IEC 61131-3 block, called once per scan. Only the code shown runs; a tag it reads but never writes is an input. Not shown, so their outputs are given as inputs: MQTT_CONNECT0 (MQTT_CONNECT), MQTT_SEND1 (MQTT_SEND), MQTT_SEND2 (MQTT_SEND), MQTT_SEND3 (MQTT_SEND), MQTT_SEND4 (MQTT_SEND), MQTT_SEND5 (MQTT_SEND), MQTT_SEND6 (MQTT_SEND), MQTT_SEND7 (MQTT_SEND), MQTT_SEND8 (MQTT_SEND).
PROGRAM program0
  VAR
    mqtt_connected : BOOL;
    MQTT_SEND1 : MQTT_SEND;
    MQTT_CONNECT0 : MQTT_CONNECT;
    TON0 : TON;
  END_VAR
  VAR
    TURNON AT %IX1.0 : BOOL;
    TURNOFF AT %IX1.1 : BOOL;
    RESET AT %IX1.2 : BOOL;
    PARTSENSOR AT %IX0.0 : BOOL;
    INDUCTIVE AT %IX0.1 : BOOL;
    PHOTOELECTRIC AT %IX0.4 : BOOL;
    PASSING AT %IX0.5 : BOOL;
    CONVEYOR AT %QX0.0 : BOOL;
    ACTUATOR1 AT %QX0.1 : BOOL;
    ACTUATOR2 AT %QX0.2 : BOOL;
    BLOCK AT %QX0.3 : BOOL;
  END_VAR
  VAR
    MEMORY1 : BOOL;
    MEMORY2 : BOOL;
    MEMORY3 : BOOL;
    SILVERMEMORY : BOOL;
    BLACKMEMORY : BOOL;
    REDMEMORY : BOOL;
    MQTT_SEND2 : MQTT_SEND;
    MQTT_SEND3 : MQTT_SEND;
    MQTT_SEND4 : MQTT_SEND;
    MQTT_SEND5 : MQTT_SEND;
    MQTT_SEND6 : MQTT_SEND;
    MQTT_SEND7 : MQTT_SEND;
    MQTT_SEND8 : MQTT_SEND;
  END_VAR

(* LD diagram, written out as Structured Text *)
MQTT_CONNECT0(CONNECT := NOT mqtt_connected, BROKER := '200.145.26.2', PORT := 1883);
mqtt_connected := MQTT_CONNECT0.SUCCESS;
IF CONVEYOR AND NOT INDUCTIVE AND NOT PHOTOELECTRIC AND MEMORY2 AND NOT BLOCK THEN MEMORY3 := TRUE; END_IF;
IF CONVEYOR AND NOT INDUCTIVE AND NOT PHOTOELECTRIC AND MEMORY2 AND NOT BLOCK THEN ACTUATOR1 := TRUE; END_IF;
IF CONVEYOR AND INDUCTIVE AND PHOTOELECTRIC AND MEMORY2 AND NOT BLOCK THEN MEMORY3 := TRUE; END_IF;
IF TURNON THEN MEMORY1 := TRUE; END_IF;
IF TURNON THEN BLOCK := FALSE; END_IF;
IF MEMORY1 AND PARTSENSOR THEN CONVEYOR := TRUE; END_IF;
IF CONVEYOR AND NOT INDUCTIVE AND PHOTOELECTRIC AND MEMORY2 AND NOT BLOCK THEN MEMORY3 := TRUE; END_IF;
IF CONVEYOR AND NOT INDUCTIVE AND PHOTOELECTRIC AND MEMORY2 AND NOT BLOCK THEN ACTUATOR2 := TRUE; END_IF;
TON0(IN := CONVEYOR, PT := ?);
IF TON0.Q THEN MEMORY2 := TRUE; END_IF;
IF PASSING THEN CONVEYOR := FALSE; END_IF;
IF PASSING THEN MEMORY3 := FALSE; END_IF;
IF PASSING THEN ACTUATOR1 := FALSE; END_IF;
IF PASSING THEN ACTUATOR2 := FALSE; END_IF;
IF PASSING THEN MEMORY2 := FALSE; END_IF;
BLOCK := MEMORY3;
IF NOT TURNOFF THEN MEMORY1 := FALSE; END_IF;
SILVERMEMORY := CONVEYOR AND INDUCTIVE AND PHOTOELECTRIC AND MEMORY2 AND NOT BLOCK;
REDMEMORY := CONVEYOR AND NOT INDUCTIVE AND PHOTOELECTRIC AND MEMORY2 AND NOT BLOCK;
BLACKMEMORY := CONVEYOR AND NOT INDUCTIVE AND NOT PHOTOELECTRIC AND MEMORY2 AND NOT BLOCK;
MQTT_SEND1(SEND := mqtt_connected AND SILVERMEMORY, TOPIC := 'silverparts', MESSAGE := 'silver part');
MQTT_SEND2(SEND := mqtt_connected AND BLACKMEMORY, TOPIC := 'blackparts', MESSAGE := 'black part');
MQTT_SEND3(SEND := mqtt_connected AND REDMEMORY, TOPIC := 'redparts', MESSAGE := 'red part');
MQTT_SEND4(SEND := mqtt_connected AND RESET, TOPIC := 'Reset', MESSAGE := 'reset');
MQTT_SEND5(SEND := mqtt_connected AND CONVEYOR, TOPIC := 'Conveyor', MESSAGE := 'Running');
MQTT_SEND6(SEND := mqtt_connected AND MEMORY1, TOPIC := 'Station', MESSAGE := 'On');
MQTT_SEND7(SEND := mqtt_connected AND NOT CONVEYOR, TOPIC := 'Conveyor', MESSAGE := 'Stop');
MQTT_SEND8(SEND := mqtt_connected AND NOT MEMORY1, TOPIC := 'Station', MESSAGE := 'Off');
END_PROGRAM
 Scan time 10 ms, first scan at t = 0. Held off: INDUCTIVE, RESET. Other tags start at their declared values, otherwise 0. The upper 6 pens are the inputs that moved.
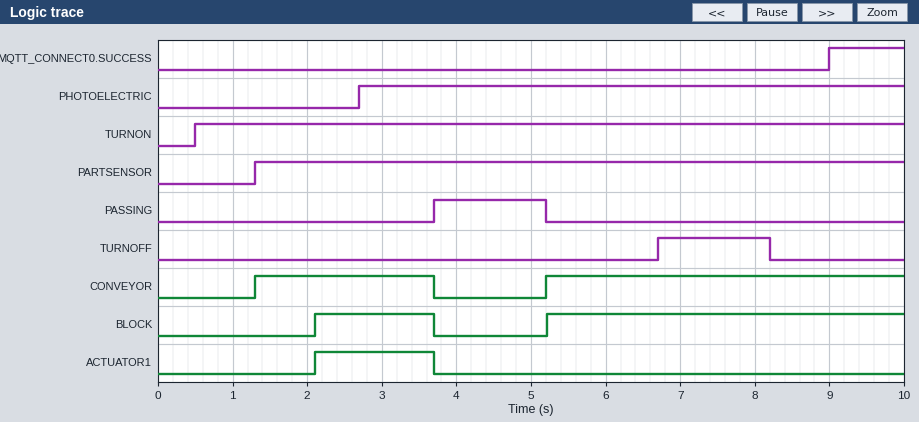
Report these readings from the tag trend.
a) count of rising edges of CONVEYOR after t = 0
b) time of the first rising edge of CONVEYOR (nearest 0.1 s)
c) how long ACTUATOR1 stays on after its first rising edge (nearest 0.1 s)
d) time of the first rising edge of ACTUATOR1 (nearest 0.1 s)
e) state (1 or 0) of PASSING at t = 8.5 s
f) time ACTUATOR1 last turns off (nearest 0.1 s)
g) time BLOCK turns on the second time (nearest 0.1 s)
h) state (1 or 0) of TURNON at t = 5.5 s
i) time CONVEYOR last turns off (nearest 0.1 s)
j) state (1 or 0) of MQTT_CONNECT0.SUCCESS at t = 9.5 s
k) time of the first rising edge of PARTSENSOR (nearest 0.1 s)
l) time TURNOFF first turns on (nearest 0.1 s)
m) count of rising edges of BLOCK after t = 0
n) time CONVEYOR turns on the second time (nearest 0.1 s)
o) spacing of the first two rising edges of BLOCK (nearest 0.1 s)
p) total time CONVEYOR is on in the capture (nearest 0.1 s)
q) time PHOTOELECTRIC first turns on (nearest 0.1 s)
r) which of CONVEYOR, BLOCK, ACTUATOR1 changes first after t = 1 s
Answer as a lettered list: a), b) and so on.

a) 2
b) 1.3 s
c) 1.6 s
d) 2.1 s
e) 0
f) 3.7 s
g) 5.2 s
h) 1
i) 3.7 s
j) 1
k) 1.3 s
l) 6.7 s
m) 2
n) 5.2 s
o) 3.1 s
p) 7.2 s
q) 2.7 s
r) CONVEYOR
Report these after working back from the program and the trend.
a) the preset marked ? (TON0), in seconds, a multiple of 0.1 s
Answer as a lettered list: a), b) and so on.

a) 0.8 s
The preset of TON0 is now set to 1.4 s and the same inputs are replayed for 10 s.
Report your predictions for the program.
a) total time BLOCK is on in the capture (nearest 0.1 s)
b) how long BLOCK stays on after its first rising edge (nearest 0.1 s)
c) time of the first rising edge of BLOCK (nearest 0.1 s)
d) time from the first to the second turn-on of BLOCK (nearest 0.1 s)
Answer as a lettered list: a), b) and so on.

a) 5.8 s
b) 1.0 s
c) 2.7 s
d) 2.5 s
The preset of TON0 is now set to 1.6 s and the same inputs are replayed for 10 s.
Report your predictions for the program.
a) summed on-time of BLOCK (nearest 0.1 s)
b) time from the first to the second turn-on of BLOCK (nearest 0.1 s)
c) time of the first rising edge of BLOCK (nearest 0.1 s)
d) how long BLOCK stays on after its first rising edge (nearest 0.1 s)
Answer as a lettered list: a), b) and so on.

a) 5.6 s
b) 2.3 s
c) 2.9 s
d) 0.8 s
